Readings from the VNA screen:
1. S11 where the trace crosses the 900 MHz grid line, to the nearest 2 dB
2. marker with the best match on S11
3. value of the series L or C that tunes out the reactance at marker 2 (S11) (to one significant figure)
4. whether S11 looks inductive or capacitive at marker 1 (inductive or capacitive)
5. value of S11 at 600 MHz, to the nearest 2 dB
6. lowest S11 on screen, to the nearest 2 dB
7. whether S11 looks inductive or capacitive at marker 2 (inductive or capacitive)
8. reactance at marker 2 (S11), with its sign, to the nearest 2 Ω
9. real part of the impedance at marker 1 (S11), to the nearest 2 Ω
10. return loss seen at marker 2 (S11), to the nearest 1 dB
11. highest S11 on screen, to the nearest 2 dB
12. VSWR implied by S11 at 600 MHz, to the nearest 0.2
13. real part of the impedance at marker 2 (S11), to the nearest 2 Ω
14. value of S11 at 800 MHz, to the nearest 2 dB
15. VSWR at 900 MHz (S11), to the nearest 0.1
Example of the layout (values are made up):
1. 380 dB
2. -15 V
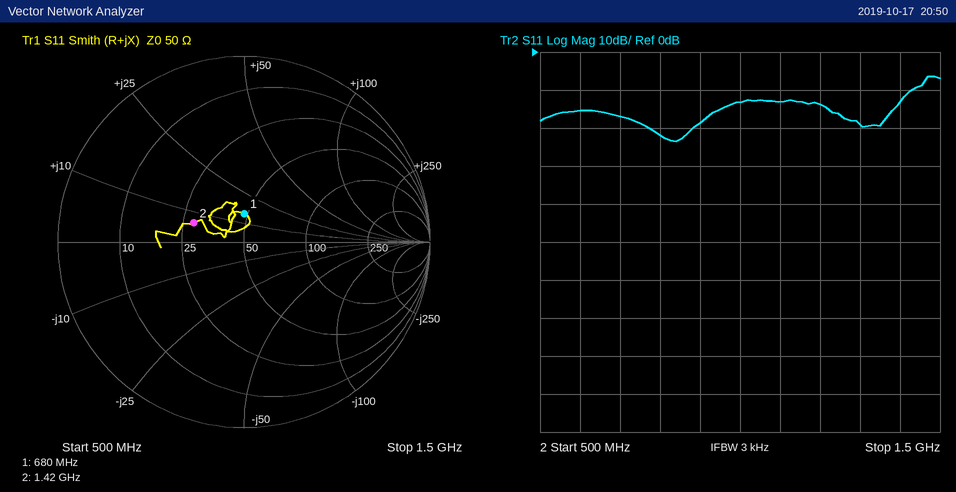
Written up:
1. -18 dB
2. marker 1
3. 20 pF
4. inductive
5. -16 dB
6. -24 dB
7. inductive
8. +6 Ω
9. 48 Ω
10. 11 dB
11. -6 dB
12. 1.4
13. 28 Ω
14. -22 dB
15. 1.3
